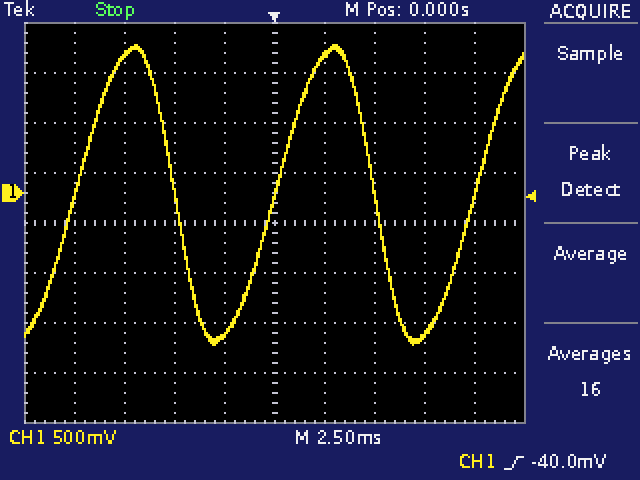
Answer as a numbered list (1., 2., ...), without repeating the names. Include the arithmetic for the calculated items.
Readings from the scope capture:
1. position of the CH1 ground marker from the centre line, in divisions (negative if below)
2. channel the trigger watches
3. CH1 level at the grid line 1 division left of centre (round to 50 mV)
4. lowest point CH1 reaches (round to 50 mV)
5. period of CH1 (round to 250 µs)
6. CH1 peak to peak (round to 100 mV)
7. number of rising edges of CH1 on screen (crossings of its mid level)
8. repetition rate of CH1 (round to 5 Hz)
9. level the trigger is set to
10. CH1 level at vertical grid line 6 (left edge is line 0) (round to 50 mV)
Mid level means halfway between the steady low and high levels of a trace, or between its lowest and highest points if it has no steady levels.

1. +0.6 div
2. CH1
3. -1.40 V
4. -1.50 V
5. 10.00 ms
6. 3.00 V
7. 3
8. 1 / 10.00 ms ≈ 100 Hz
9. -40.0 mV
10. 1.35 V
